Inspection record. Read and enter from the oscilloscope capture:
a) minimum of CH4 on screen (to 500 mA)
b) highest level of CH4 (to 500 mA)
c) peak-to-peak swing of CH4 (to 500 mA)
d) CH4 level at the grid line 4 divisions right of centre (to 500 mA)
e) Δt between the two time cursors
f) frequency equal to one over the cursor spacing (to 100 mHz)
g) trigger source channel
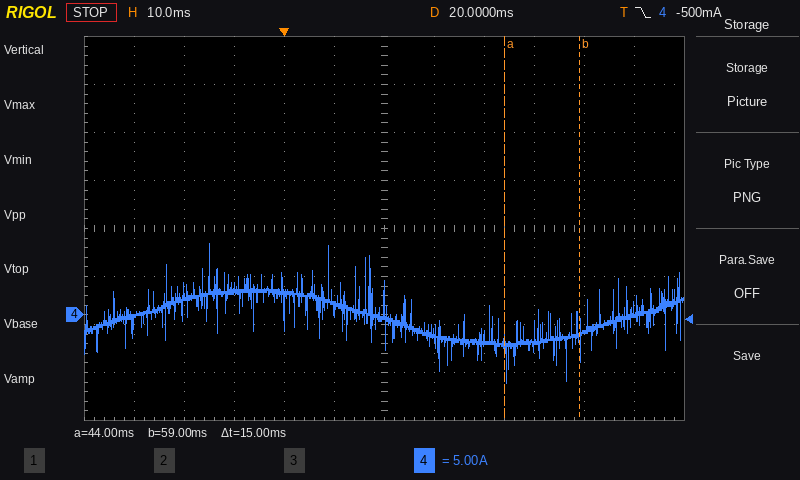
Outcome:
-7.0 A
7.5 A
14.5 A
-1.5 A
15 ms
66.7 Hz
CH4
